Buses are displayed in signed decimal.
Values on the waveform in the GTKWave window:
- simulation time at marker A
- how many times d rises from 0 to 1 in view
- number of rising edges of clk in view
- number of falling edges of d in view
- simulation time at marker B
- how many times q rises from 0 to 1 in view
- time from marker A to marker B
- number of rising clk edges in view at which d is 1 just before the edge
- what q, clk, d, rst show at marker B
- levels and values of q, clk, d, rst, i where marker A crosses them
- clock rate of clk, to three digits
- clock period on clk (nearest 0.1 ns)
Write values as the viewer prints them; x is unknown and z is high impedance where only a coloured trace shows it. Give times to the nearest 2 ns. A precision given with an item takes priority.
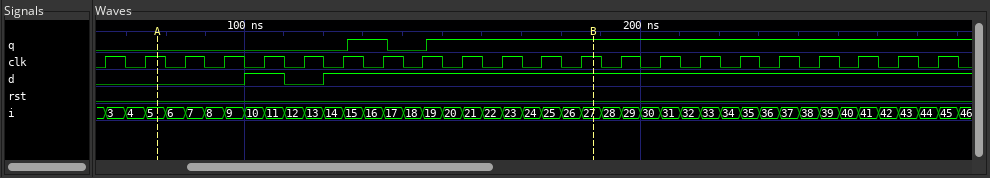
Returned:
78 ns
2
22
1
188 ns
2
110 ns
17
q=1, clk=1, d=1, rst=0
q=0, clk=1, d=0, rst=0, i=5
100 MHz
10 ns
